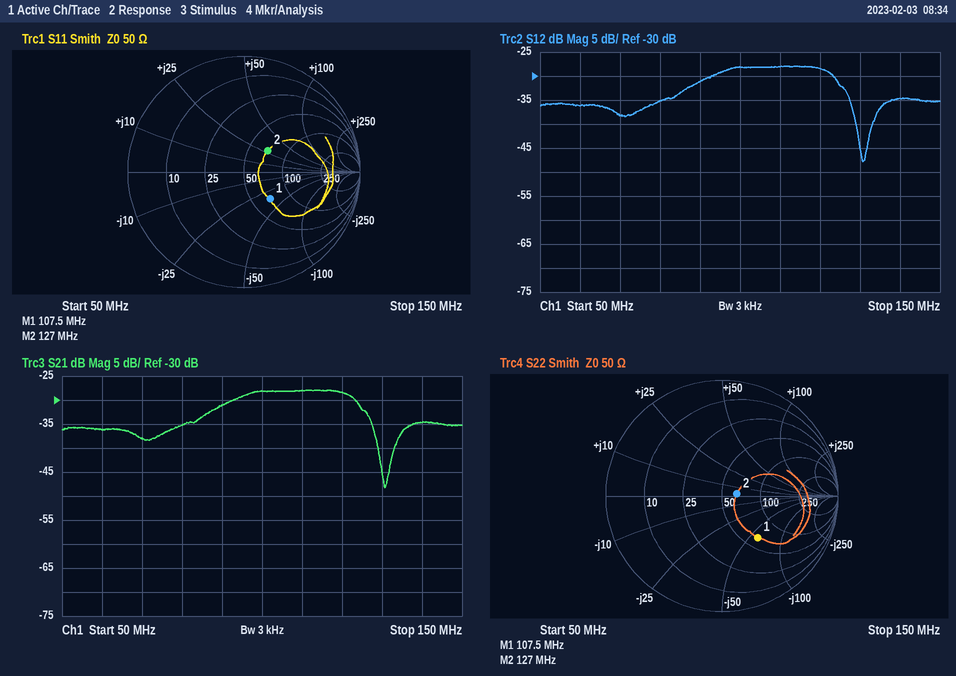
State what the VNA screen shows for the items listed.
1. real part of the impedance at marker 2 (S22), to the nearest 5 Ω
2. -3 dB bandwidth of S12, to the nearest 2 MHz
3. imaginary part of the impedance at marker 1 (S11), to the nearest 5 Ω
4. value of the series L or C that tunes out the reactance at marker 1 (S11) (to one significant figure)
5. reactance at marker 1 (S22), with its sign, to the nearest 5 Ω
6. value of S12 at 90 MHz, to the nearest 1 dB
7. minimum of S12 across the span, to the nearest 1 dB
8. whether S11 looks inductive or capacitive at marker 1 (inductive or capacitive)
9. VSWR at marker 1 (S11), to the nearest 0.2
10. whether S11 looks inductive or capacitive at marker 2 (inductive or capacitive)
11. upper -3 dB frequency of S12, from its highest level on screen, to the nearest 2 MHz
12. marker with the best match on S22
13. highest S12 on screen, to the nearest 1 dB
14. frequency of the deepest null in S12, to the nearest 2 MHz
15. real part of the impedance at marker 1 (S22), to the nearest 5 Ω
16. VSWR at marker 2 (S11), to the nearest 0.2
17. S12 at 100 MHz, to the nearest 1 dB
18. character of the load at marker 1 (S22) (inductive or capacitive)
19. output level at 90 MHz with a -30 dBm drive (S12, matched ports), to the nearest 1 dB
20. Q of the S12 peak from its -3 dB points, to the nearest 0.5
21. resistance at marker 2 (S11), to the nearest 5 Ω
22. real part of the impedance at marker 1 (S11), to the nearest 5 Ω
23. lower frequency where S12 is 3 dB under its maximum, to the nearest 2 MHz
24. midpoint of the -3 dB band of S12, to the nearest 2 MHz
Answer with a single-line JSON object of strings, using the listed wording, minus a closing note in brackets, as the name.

{"real part of the impedance at marker 2 (S22), to the nearest 5 Ω": "65 Ω", "-3 dB bandwidth of S12, to the nearest 2 MHz": "34 MHz", "imaginary part of the impedance at marker 1 (S11), to the nearest 5 Ω": "-35 Ω", "value of the series L or C that tunes out the reactance at marker 1 (S11)": "50 nH", "reactance at marker 1 (S22), with its sign, to the nearest 5 Ω": "-60 Ω", "value of S12 at 90 MHz, to the nearest 1 dB": "-31 dB", "minimum of S12 across the span, to the nearest 1 dB": "-48 dB", "whether S11 looks inductive or capacitive at marker 1": "capacitive", "VSWR at marker 1 (S11), to the nearest 0.2": "2.0", "whether S11 looks inductive or capacitive at marker 2": "inductive", "upper -3 dB frequency of S12, from its highest level on screen, to the nearest 2 MHz": "124 MHz", "marker with the best match on S22": "marker 2", "highest S12 on screen, to the nearest 1 dB": "-28 dB", "frequency of the deepest null in S12, to the nearest 2 MHz": "130 MHz", "real part of the impedance at marker 1 (S22), to the nearest 5 Ω": "65 Ω", "VSWR at marker 2 (S11), to the nearest 0.2": "1.8", "S12 at 100 MHz, to the nearest 1 dB": "-28 dB", "character of the load at marker 1 (S22)": "capacitive", "output level at 90 MHz with a -30 dBm drive (S12, matched ports), to the nearest 1 dB": "-61 dBm", "Q of the S12 peak from its -3 dB points, to the nearest 0.5": "3.0", "resistance at marker 2 (S11), to the nearest 5 Ω": "70 Ω", "real part of the impedance at marker 1 (S11), to the nearest 5 Ω": "70 Ω", "lower frequency where S12 is 3 dB under its maximum, to the nearest 2 MHz": "90 MHz", "midpoint of the -3 dB band of S12, to the nearest 2 MHz": "108 MHz"}
